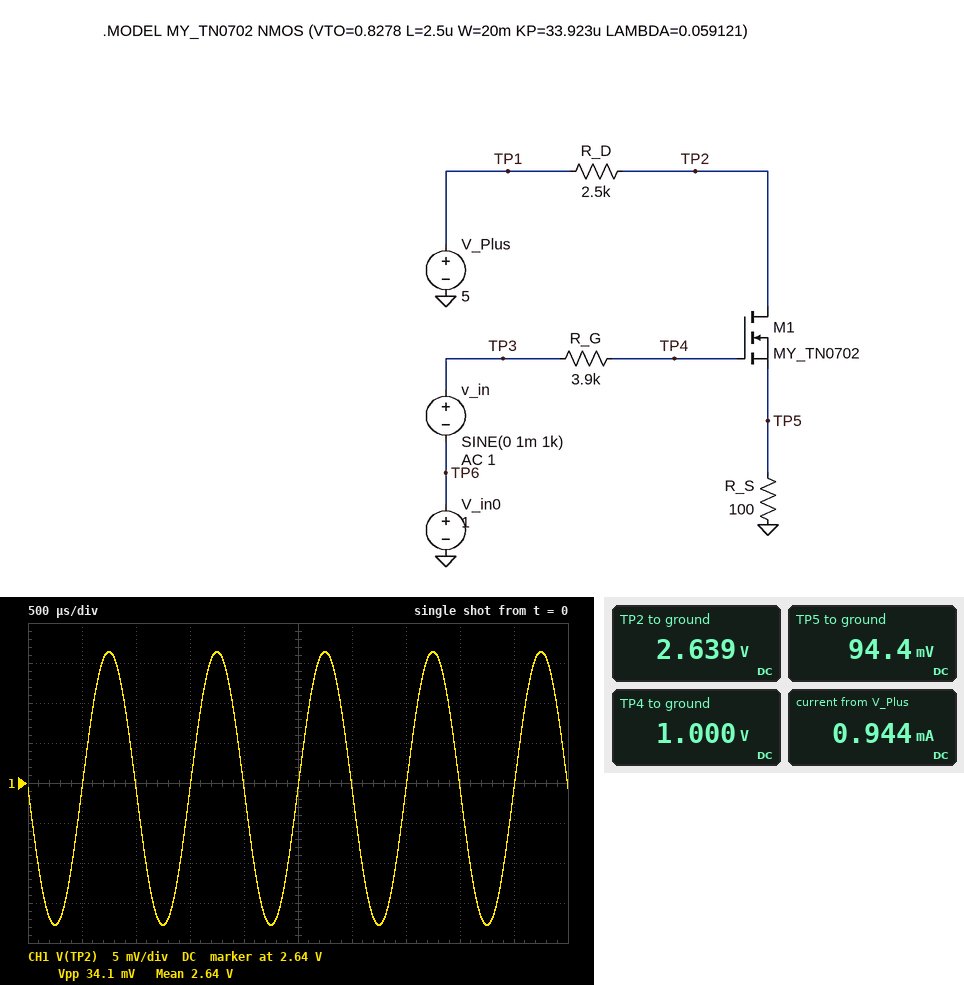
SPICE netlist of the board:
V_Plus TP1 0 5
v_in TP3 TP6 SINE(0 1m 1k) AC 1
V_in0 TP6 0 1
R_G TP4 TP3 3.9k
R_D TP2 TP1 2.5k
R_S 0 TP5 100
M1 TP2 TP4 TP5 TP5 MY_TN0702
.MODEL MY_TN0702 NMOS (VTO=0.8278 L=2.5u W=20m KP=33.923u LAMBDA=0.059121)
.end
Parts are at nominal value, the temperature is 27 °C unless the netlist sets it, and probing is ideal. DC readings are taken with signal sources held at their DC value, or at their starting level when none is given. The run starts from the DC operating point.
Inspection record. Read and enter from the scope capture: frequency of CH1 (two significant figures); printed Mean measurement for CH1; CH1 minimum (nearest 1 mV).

1.0 kHz
2.64 V
2.622 V
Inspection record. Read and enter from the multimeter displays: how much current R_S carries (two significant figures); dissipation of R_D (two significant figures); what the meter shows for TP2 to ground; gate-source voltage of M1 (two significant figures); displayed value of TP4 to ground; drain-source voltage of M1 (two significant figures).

940 µA
2.2 mW
2.639 V
910 mV
1.000 V
2.5 V
